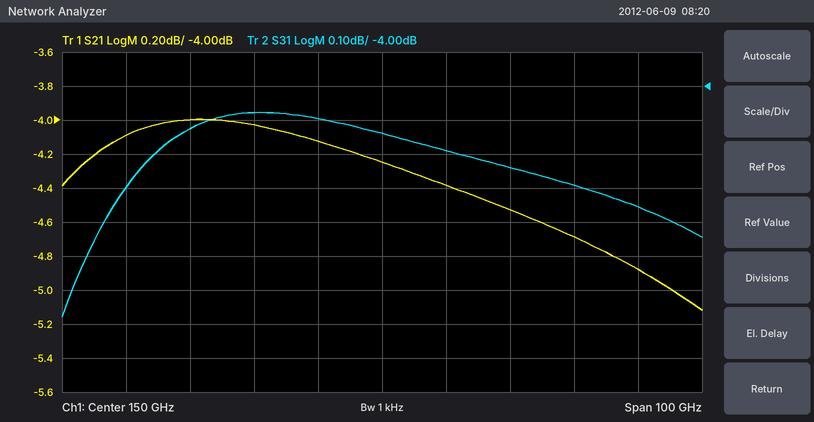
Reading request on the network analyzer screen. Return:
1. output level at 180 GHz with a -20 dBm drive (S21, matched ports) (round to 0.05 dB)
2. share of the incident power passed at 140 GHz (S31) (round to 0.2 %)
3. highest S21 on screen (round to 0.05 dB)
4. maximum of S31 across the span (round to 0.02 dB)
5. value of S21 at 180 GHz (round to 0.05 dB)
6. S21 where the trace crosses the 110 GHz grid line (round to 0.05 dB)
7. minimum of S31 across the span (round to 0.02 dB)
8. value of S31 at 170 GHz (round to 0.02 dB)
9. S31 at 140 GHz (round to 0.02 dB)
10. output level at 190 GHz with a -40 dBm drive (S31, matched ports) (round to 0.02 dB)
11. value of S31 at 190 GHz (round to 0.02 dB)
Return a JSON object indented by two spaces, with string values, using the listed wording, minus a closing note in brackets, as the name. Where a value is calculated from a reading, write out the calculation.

{
  "output level at 180 GHz with a -20 dBm drive (S21, matched ports)": "-20 dBm + (-4.70 dB) = -24.70 dBm",
  "share of the incident power passed at 140 GHz (S31)": "10^(-4.1/10) ≈ 38.9 %, so 39.0 % to the nearest 0.2 %",
  "highest S21 on screen": "-4.00 dB",
  "maximum of S31 across the span": "-4.08 dB",
  "value of S21 at 180 GHz": "-4.70 dB",
  "S21 where the trace crosses the 110 GHz grid line": "-4.10 dB",
  "minimum of S31 across the span": "-4.68 dB",
  "value of S31 at 170 GHz": "-4.24 dB",
  "S31 at 140 GHz": "-4.10 dB",
  "output level at 190 GHz with a -40 dBm drive (S31, matched ports)": "-40 dBm + (-4.36 dB) = -44.36 dBm",
  "value of S31 at 190 GHz": "-4.36 dB"
}
